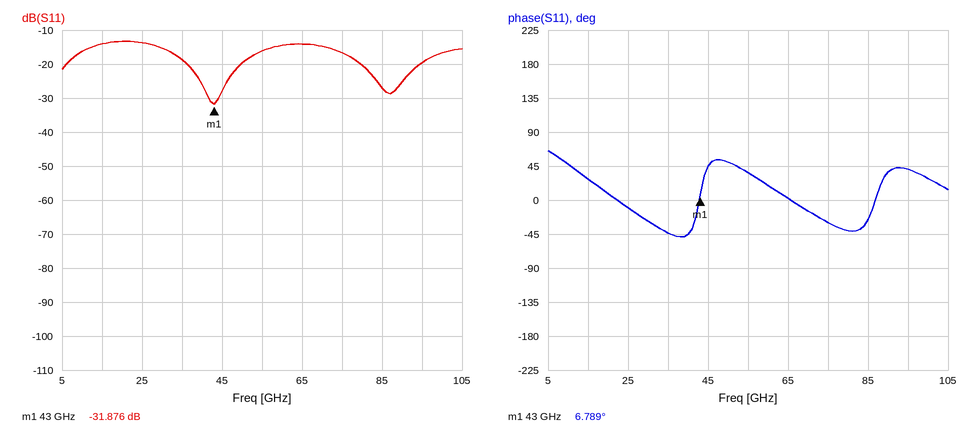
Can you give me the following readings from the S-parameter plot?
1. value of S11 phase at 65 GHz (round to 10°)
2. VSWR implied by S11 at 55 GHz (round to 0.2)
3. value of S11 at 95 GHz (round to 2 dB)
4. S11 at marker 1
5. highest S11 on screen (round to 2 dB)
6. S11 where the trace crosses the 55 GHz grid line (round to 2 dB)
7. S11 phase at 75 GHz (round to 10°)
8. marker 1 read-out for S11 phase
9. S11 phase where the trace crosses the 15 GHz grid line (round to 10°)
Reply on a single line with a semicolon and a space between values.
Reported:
0°; 1.4; -20 dB; -31.876 dB; -14 dB; -16 dB; -30°; 6.789°; 30°
